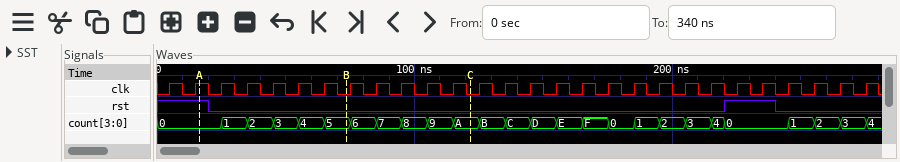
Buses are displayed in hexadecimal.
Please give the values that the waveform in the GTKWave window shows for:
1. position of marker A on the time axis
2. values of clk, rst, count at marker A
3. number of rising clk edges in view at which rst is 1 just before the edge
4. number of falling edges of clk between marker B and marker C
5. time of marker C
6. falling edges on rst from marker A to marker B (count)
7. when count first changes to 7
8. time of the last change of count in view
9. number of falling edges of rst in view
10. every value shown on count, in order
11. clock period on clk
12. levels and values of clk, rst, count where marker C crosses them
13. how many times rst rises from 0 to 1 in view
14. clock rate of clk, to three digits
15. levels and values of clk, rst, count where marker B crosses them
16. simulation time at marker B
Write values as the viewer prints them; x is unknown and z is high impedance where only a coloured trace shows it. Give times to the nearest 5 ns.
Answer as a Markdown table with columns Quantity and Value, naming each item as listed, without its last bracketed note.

| Quantity | Value |
|---|---|
| position of marker A on the time axis | 15 ns |
| values of clk, rst, count at marker A | clk=1, rst=1, count=0 |
| number of rising clk edges in view at which rst is 1 just before the edge | 4 |
| number of falling edges of clk between marker B and marker C | 5 |
| time of marker C | 120 ns |
| falling edges on rst from marker A to marker B | 1 |
| when count first changes to 7 | 85 ns |
| time of the last change of count in view | 275 ns |
| number of falling edges of rst in view | 2 |
| every value shown on count, in order | 0, 1, 2, 3, 4, 5, 6, 7, 8, 9, A, B, C, D, E, F, 0, 1, 2, 3, 4, 0, 1, 2, 3, 4 |
| clock period on clk | 10 ns |
| levels and values of clk, rst, count where marker C crosses them | clk=0, rst=0, count=A |
| how many times rst rises from 0 to 1 in view | 1 |
| clock rate of clk, to three digits | 100 MHz |
| levels and values of clk, rst, count where marker B crosses them | clk=0, rst=0, count=5 |
| simulation time at marker B | 75 ns |
